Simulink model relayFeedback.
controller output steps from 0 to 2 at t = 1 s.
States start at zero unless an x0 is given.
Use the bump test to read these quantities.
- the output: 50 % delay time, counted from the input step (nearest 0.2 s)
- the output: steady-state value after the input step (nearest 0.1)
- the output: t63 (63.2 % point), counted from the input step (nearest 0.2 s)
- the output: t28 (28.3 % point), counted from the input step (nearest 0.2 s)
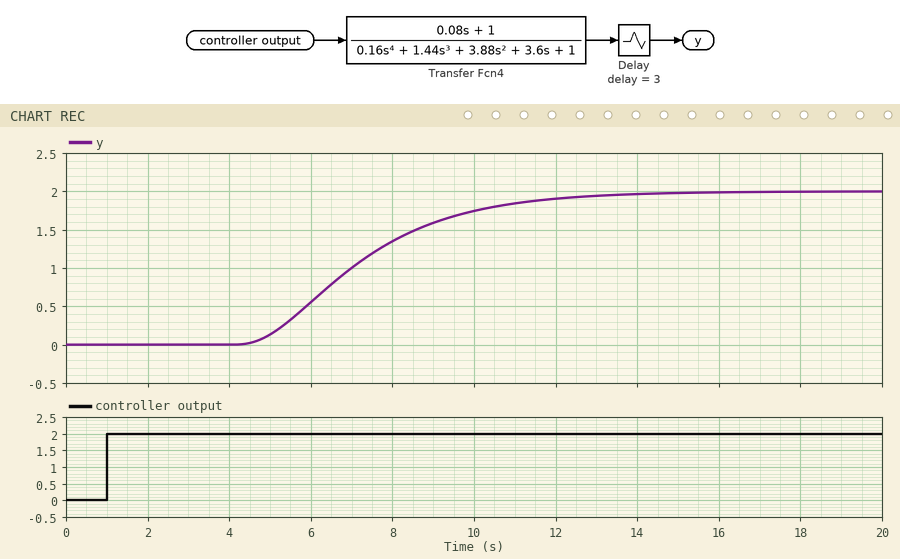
6.0 s
2.0
6.8 s
5.0 s
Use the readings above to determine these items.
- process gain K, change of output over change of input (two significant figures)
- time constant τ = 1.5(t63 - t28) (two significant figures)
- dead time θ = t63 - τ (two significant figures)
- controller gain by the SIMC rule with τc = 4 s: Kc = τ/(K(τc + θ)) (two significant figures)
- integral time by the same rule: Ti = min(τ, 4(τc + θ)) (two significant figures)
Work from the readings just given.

1.0
2.7 s
4.1 s
0.33
2.7 s
